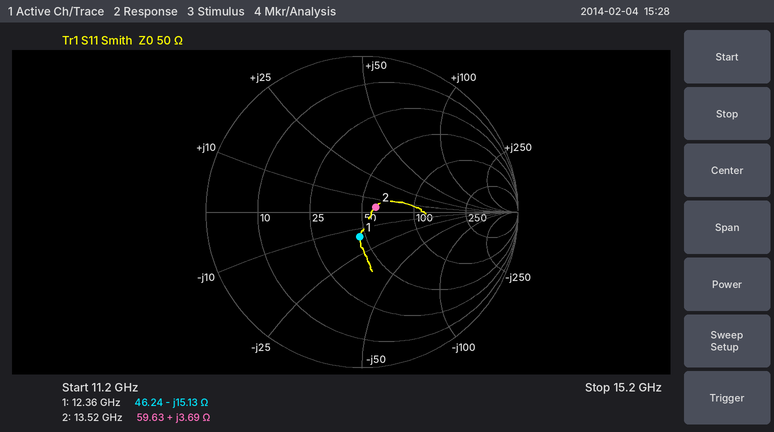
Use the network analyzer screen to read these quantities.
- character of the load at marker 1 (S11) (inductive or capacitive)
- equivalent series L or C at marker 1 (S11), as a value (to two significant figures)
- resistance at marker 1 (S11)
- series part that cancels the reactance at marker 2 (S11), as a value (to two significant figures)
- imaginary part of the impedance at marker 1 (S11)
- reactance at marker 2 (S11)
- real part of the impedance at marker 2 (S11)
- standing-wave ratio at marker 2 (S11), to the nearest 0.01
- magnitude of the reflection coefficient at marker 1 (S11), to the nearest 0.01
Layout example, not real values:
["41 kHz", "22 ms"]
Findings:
["capacitive", "850 fF", "46.24 Ω", "3.2 pF", "-15.13 Ω", "+3.69 Ω", "59.63 Ω", "1.21", "0.16"]
